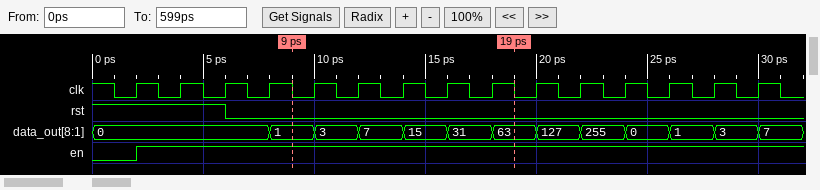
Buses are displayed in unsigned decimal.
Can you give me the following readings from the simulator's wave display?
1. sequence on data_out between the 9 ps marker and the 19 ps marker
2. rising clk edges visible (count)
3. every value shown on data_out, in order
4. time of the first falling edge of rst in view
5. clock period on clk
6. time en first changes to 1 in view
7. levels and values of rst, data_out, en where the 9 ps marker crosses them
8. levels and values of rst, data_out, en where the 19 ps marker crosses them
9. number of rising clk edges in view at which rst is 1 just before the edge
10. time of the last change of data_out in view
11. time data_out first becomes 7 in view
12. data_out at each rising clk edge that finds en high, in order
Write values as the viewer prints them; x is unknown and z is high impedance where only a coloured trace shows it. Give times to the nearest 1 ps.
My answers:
1, 3, 7, 15, 31, 63
15
0, 1, 3, 7, 15, 31, 63, 127, 255, 0, 1, 3, 7
6 ps
2 ps
2 ps
rst=0, data_out=1, en=1
rst=0, data_out=63, en=1
3
30 ps
12 ps
0, 0, 0, 1, 3, 7, 15, 31, 63, 127, 255, 0, 1, 3
